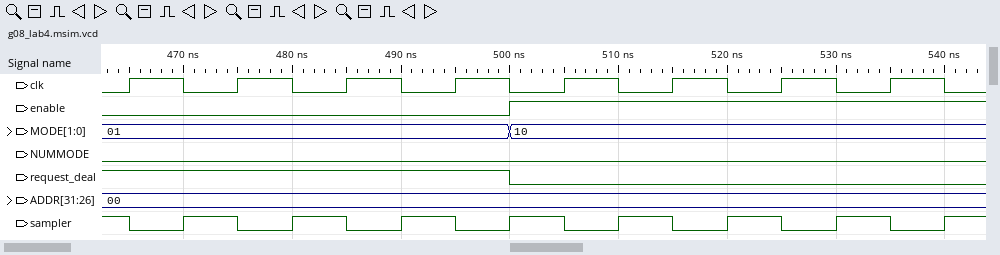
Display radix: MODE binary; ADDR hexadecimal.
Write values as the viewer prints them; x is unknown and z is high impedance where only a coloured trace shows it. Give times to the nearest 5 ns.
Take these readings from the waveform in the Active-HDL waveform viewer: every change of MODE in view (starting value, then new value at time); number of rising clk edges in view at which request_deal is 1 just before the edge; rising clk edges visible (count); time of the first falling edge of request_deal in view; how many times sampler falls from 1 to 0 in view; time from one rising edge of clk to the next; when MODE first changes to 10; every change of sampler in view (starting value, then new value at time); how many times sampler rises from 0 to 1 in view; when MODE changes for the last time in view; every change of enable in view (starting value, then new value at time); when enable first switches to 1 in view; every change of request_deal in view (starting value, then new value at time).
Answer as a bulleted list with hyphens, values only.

- 01, 10 at 500 ns
- 4
- 8
- 500 ns
- 8
- 10 ns
- 500 ns
- 1, 0 at 465 ns, 1 at 470 ns, 0 at 475 ns, 1 at 480 ns, 0 at 485 ns, 1 at 490 ns, 0 at 495 ns, 1 at 500 ns, 0 at 505 ns, 1 at 510 ns, 0 at 515 ns, 1 at 520 ns, 0 at 525 ns, 1 at 530 ns, 0 at 535 ns, 1 at 540 ns
- 8
- 500 ns
- 0, 1 at 500 ns
- 500 ns
- 1, 0 at 500 ns
